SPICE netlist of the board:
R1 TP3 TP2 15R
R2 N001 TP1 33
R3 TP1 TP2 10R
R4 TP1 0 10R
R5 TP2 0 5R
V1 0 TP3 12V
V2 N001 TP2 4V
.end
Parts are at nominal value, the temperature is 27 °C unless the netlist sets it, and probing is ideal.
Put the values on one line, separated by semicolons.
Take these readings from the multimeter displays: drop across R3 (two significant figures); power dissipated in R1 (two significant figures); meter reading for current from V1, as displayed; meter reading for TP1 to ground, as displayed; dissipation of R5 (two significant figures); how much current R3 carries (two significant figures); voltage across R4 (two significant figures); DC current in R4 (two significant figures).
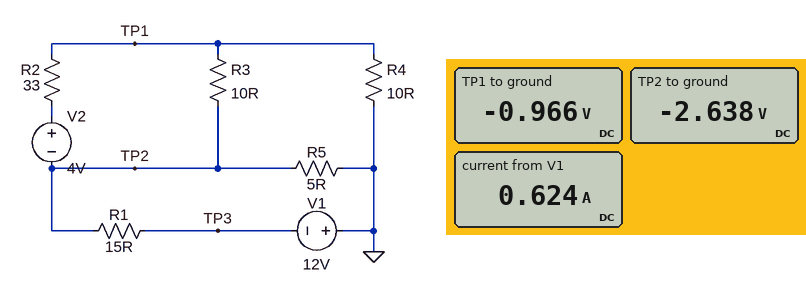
1.7 V; 5.8 W; 0.624 A; -0.966 V; 1.4 W; 170 mA; 970 mV; 97 mA
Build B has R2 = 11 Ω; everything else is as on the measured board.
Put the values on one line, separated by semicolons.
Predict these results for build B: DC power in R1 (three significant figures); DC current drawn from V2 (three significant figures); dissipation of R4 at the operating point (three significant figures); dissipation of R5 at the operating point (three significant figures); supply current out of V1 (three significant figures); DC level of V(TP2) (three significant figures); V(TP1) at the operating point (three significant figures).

5.66 W; 163 mA; 33.3 mW; 1.55 W; 614 mA; -2.78 V; -577 mV
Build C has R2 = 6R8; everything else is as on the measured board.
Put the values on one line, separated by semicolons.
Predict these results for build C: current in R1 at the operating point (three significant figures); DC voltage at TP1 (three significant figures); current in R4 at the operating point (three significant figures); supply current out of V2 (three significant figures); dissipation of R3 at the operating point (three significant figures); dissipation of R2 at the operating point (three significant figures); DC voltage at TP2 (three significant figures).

609 mA; -348 mV; 34.8 mA; 217 mA; 636 mW; 321 mW; -2.87 V
